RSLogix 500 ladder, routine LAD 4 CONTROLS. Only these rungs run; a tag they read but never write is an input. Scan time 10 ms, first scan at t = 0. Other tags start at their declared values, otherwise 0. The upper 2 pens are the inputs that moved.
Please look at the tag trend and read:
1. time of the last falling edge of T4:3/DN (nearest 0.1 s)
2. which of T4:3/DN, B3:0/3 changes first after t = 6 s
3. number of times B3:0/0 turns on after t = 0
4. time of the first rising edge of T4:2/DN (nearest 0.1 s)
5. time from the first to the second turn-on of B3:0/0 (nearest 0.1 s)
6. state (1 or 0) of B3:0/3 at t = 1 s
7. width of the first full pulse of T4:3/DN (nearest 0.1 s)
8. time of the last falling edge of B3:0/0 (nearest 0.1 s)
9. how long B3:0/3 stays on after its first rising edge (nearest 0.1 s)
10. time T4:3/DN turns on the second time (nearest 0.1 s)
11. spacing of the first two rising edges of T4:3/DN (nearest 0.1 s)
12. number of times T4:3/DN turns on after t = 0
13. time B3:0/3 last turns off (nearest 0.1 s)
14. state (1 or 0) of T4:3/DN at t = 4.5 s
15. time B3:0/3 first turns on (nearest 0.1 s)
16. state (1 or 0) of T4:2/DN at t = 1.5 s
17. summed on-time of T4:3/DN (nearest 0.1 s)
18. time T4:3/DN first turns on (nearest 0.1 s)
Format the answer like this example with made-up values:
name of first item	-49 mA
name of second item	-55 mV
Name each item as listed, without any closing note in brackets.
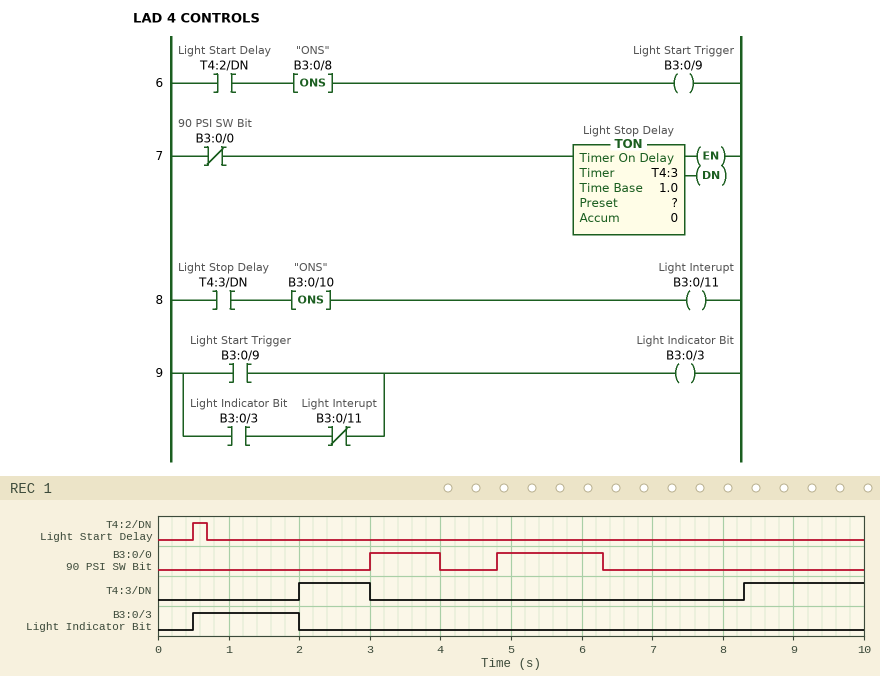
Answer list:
time of the last falling edge of T4:3/DN	3.0 s
which of T4:3/DN, B3:0/3 changes first after t = 6 s	T4:3/DN
number of times B3:0/0 turns on after t = 0	2
time of the first rising edge of T4:2/DN	0.5 s
time from the first to the second turn-on of B3:0/0	1.8 s
state (1 or 0) of B3:0/3 at t = 1 s	1
width of the first full pulse of T4:3/DN	1.0 s
time of the last falling edge of B3:0/0	6.3 s
how long B3:0/3 stays on after its first rising edge	1.5 s
time T4:3/DN turns on the second time	8.3 s
spacing of the first two rising edges of T4:3/DN	6.3 s
number of times T4:3/DN turns on after t = 0	2
time B3:0/3 last turns off	2.0 s
state (1 or 0) of T4:3/DN at t = 4.5 s	0
time B3:0/3 first turns on	0.5 s
state (1 or 0) of T4:2/DN at t = 1.5 s	0
summed on-time of T4:3/DN	2.7 s
time T4:3/DN first turns on	2.0 s
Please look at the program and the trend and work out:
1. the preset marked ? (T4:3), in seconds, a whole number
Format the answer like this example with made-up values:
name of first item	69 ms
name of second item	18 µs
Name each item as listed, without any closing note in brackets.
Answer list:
the preset marked ? (T4:3), in seconds, a whole number	2 s
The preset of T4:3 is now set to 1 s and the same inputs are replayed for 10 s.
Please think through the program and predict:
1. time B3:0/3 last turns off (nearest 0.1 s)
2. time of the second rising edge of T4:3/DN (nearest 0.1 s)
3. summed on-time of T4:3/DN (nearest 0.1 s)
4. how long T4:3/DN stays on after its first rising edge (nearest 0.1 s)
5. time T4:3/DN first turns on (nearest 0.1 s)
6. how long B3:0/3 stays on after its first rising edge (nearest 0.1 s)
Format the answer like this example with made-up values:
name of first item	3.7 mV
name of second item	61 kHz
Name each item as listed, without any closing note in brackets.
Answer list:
time B3:0/3 last turns off	1.0 s
time of the second rising edge of T4:3/DN	7.3 s
summed on-time of T4:3/DN	4.7 s
how long T4:3/DN stays on after its first rising edge	2.0 s
time T4:3/DN first turns on	1.0 s
how long B3:0/3 stays on after its first rising edge	0.5 s
